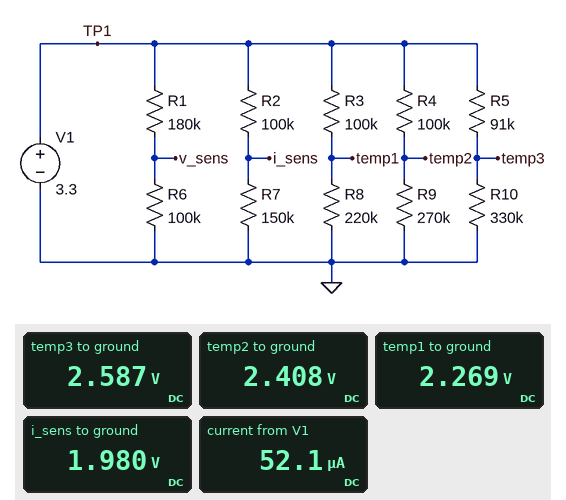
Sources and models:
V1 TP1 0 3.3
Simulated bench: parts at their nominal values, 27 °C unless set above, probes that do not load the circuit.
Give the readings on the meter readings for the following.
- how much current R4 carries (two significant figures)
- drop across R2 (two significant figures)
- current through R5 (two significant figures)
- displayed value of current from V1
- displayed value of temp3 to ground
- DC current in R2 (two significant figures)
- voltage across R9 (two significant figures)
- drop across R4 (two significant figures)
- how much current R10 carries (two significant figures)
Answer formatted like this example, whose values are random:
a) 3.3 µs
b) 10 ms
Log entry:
a) 8.9 µA
b) 1.3 V
c) 7.8 µA
d) 52.1 µA
e) 2.587 V
f) 13 µA
g) 2.4 V
h) 890 mV
i) 7.8 µA
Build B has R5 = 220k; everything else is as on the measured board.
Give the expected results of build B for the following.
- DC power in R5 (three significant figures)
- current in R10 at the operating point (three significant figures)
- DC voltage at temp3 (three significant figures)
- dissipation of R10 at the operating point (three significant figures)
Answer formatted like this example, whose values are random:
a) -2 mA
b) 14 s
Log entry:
a) 7.92 µW
b) 6.00 µA
c) 1.98 V
d) 11.9 µW
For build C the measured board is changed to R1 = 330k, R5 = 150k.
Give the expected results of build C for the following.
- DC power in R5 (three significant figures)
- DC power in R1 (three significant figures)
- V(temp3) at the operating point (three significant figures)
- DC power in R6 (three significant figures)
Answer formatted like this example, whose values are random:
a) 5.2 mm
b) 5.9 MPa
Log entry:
a) 7.09 µW
b) 19.4 µW
c) 2.27 V
d) 5.89 µW
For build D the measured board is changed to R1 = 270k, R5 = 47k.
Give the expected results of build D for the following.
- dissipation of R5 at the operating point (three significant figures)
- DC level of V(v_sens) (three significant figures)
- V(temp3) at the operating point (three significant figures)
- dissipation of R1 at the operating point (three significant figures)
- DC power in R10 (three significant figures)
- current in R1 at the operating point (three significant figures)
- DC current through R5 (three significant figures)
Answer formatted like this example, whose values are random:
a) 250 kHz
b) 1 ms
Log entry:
a) 3.60 µW
b) 892 mV
c) 2.89 V
d) 21.5 µW
e) 25.3 µW
f) 8.92 µA
g) 8.75 µA
